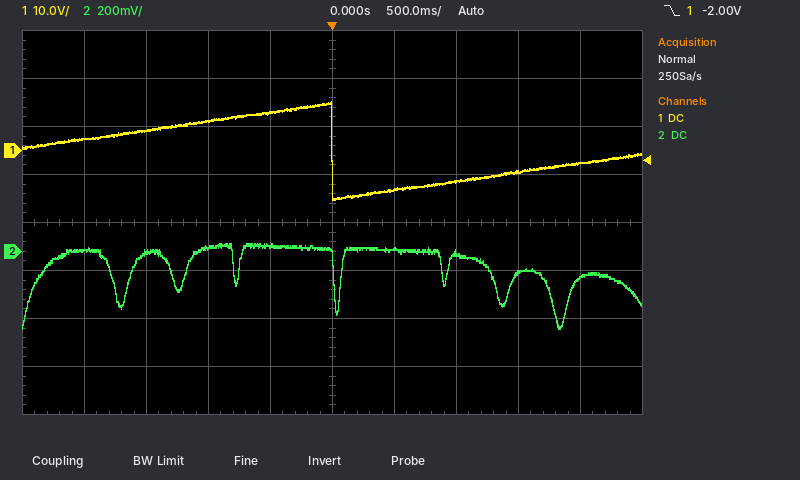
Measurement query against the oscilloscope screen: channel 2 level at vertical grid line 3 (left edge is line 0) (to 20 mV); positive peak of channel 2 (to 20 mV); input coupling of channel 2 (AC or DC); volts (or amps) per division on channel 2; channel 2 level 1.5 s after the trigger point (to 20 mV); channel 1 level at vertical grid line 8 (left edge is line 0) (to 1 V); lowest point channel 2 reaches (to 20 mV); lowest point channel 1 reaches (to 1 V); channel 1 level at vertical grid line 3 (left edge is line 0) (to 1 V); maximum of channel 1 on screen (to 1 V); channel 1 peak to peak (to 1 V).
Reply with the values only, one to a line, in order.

20 mV
40 mV
DC
200 mV
-100 mV
-4 V
-320 mV
-10 V
6 V
10 V
20 V
